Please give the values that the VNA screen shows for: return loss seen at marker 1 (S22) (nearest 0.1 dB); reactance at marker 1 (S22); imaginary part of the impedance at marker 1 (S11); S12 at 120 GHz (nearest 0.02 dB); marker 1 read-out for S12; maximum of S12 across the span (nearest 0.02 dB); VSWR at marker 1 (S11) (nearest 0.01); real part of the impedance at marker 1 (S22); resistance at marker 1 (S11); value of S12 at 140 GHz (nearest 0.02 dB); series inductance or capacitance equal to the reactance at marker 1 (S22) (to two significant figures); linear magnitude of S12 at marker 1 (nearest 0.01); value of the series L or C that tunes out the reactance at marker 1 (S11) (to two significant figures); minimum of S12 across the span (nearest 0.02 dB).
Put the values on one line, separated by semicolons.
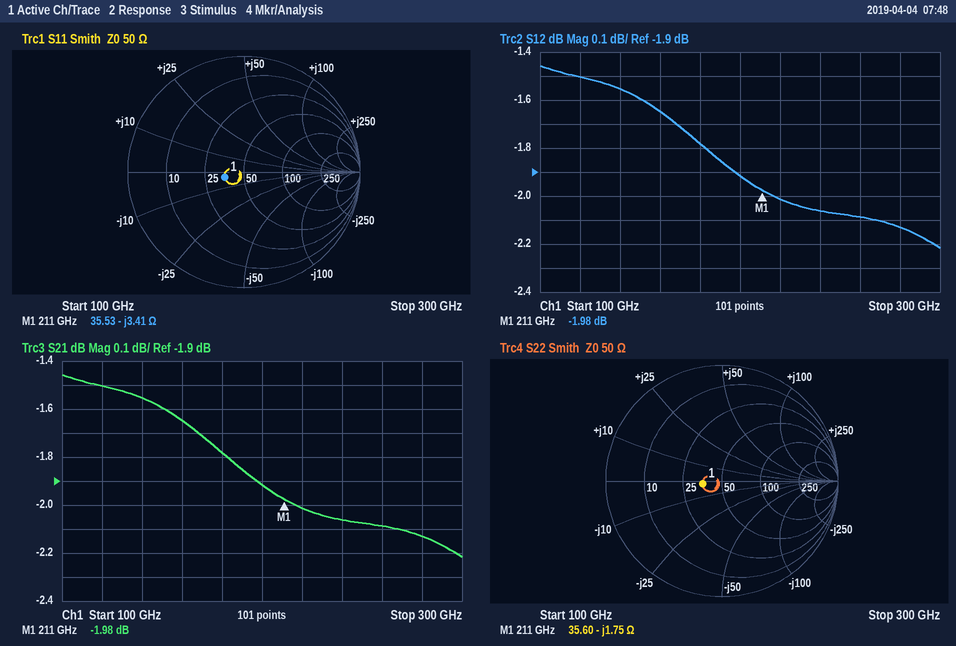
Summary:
15.4 dB; -1.75 Ω; -3.41 Ω; -1.50 dB; -1.98 dB; -1.46 dB; 1.42; 35.60 Ω; 35.53 Ω; -1.56 dB; 430 fF; 0.80; 2.6 pH; -2.22 dB
